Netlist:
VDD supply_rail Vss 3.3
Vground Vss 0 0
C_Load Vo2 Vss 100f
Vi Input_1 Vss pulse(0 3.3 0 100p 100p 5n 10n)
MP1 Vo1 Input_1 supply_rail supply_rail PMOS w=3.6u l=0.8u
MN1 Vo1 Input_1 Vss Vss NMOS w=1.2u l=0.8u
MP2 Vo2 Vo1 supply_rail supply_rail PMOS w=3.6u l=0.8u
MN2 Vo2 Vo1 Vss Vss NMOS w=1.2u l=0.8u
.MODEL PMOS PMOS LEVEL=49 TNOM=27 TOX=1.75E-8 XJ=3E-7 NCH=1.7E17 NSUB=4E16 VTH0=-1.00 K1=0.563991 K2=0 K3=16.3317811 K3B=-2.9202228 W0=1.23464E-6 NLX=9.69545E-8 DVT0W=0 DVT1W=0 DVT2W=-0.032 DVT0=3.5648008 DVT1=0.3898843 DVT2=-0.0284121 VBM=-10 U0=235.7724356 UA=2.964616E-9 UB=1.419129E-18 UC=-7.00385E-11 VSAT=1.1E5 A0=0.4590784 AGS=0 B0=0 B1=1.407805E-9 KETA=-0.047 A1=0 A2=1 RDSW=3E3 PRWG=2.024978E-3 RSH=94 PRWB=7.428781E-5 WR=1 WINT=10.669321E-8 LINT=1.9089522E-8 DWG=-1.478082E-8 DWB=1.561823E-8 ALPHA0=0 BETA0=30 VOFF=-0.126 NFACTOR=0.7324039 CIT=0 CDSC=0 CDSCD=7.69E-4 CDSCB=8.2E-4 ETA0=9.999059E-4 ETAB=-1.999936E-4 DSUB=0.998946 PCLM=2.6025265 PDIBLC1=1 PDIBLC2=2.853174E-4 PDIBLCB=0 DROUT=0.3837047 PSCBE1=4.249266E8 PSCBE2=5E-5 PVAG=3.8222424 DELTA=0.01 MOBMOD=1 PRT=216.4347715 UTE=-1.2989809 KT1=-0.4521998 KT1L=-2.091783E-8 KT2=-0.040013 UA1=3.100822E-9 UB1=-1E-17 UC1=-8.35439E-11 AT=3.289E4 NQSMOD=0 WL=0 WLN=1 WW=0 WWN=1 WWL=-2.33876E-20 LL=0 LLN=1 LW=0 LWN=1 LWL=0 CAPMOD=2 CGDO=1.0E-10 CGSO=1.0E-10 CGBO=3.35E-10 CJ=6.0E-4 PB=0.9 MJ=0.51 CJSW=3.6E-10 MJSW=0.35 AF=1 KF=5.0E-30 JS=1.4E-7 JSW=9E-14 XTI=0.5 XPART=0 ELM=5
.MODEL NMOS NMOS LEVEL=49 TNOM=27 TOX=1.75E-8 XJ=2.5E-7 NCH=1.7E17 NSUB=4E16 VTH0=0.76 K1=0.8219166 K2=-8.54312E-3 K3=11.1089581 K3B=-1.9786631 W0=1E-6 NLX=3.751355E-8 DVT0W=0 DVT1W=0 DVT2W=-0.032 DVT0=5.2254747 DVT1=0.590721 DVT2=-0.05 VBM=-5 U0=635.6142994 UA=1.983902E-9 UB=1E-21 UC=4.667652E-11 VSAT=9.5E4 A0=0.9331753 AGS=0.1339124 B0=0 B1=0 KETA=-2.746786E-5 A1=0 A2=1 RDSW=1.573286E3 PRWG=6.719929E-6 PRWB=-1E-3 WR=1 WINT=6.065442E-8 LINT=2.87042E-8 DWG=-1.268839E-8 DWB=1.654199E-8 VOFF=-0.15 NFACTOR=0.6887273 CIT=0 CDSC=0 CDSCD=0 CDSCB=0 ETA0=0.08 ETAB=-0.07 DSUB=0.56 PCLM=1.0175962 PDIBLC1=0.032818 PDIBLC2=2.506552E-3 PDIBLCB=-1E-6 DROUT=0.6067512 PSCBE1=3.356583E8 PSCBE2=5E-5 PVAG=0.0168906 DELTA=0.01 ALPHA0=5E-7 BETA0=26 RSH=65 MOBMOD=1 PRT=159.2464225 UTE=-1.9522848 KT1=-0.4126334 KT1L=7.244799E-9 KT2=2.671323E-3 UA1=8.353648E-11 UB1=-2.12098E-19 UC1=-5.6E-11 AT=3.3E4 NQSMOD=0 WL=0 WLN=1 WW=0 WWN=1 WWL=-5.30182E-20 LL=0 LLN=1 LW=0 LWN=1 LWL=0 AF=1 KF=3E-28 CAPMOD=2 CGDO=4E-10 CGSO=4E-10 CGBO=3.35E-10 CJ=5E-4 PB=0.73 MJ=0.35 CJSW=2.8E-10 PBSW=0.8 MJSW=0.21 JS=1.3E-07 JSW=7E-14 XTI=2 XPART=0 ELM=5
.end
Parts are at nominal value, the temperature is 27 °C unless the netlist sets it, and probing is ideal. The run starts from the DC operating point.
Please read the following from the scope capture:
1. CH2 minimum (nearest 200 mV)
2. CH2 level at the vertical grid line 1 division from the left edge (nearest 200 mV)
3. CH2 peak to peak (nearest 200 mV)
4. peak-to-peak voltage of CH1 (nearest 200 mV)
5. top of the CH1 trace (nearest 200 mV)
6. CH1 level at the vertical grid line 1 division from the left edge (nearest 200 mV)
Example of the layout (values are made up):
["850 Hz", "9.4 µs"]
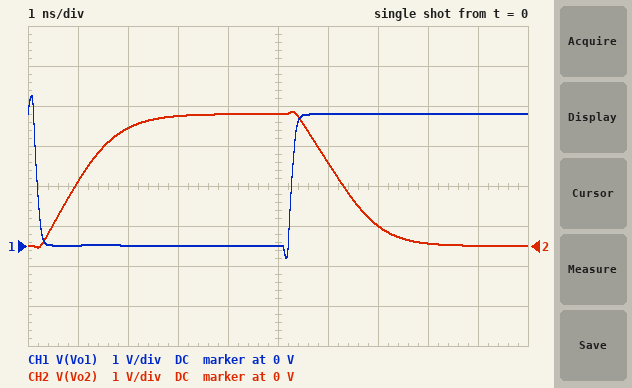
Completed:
["0 V", "1.6 V", "3.4 V", "4.0 V", "3.8 V", "0 V"]
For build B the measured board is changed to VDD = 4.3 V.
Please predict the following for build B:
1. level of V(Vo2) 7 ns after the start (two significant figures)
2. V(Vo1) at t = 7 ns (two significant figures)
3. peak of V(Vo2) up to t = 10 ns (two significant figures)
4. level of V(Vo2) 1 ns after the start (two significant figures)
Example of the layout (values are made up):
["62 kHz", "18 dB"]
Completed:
["270 mV", "4.3 V", "4.4 V", "2.6 V"]
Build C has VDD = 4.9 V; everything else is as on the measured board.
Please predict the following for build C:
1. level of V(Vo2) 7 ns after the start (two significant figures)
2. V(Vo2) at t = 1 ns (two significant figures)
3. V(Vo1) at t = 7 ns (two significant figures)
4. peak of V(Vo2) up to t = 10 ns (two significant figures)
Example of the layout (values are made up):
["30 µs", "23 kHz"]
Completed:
["200 mV", "3.0 V", "4.9 V", "5.0 V"]
